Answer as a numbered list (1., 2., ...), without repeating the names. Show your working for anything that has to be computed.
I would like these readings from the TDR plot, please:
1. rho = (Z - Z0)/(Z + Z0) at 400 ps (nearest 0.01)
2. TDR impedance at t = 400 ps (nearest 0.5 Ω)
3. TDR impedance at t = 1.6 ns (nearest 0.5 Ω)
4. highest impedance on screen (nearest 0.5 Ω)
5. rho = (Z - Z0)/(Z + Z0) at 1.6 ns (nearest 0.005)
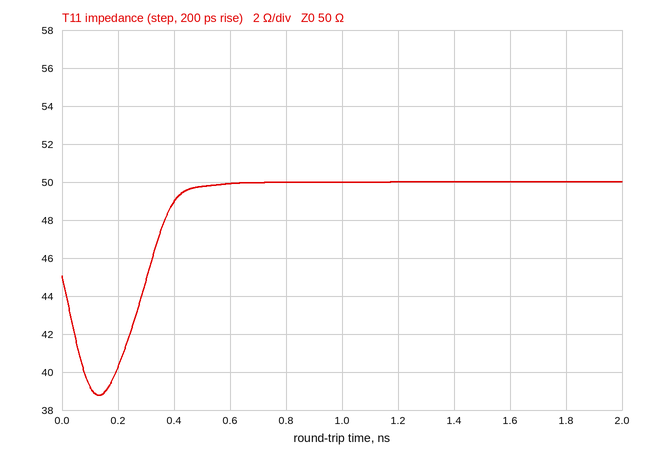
1. (49 − 50)/(49 + 50) ≈ -0.01
2. 49.0 Ω
3. 50.0 Ω
4. 50.0 Ω
5. (50 − 50)/(50 + 50) ≈ 0.000
